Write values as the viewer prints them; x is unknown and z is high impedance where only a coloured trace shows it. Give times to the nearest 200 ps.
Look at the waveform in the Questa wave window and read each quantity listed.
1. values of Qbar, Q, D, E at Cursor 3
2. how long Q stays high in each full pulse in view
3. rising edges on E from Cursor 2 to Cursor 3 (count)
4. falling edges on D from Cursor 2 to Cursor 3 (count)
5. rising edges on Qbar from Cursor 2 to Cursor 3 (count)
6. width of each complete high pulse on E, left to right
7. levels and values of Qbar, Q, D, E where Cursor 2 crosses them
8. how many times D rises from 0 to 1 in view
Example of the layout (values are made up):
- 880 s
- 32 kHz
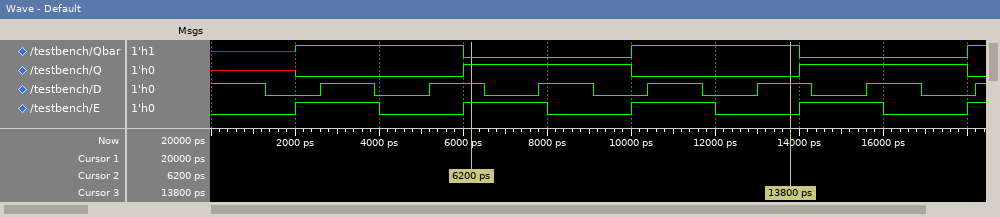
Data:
- Qbar=1, Q=0, D=1, E=0
- 4000 ps, 4000 ps
- 1
- 3
- 1
- 2000 ps, 2000 ps, 2000 ps, 2000 ps
- Qbar=0, Q=1, D=1, E=1
- 7
